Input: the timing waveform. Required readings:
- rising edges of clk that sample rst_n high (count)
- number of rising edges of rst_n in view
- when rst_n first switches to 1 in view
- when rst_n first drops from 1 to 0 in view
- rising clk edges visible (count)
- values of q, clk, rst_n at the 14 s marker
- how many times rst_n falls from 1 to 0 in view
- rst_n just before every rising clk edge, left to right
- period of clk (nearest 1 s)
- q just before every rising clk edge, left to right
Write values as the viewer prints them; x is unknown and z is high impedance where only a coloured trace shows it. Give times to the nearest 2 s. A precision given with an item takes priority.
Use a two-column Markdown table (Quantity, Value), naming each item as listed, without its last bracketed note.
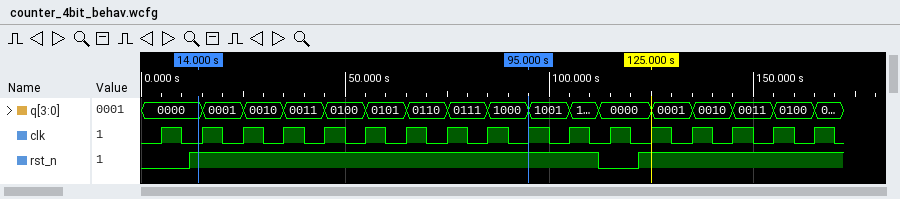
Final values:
| Quantity | Value |
|---|---|
| rising edges of clk that sample rst_n high | 15 |
| number of rising edges of rst_n in view | 2 |
| when rst_n first switches to 1 in view | 12 s |
| when rst_n first drops from 1 to 0 in view | 112 s |
| rising clk edges visible | 17 |
| values of q, clk, rst_n at the 14 s marker | q=0000, clk=0, rst_n=1 |
| how many times rst_n falls from 1 to 0 in view | 1 |
| rst_n just before every rising clk edge, left to right | 0 1 1 1 1 1 1 1 1 1 1 0 1 1 1 1 1 |
| period of clk | 10 s |
| q just before every rising clk edge, left to right | 0000, 0000, 0001, 0010, 0011, 0100, 0101, 0110, 0111, 1000, 1001, 0000, 0000, 0001, 0010, 0011, 0100 |
